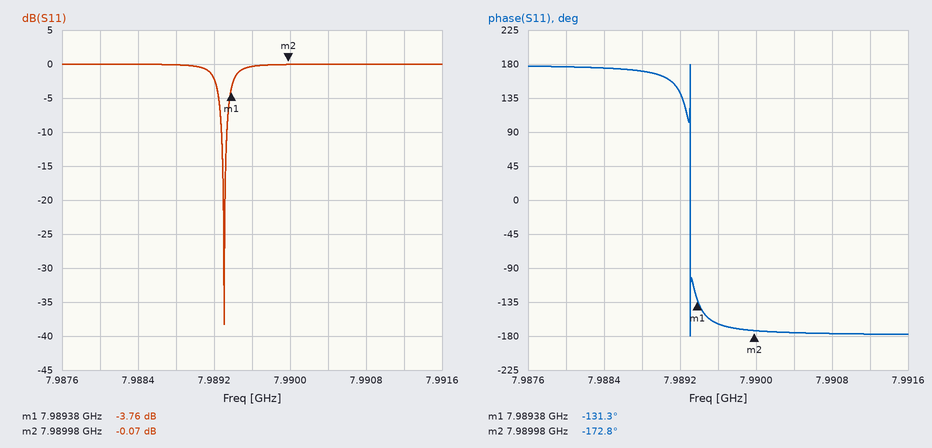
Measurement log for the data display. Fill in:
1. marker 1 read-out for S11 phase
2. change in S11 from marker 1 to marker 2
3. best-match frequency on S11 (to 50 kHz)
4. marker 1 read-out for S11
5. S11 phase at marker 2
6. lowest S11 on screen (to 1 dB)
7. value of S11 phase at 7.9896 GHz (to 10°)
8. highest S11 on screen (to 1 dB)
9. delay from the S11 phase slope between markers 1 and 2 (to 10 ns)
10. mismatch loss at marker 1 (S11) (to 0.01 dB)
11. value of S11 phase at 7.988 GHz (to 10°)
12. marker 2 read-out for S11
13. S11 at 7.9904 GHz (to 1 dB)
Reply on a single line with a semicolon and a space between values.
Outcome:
-131.3°; 3.69 dB; 7.98930 GHz; -3.76 dB; -172.8°; -38 dB; -160°; 0 dB; 190 ns; 2.37 dB; 180°; -0.07 dB; 0 dB
